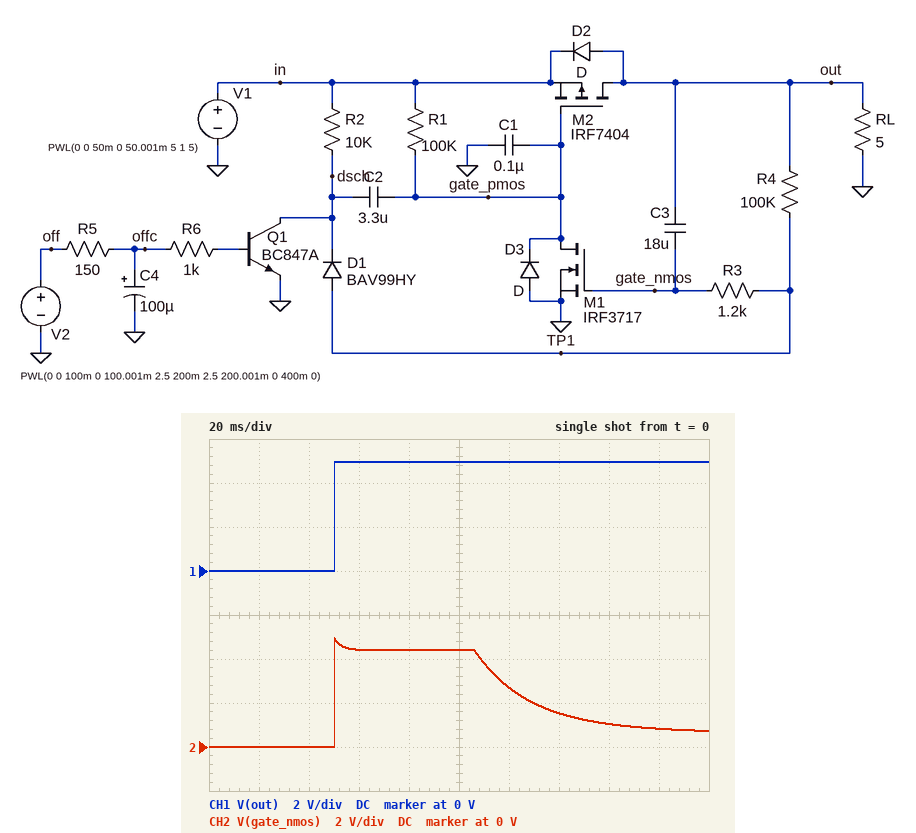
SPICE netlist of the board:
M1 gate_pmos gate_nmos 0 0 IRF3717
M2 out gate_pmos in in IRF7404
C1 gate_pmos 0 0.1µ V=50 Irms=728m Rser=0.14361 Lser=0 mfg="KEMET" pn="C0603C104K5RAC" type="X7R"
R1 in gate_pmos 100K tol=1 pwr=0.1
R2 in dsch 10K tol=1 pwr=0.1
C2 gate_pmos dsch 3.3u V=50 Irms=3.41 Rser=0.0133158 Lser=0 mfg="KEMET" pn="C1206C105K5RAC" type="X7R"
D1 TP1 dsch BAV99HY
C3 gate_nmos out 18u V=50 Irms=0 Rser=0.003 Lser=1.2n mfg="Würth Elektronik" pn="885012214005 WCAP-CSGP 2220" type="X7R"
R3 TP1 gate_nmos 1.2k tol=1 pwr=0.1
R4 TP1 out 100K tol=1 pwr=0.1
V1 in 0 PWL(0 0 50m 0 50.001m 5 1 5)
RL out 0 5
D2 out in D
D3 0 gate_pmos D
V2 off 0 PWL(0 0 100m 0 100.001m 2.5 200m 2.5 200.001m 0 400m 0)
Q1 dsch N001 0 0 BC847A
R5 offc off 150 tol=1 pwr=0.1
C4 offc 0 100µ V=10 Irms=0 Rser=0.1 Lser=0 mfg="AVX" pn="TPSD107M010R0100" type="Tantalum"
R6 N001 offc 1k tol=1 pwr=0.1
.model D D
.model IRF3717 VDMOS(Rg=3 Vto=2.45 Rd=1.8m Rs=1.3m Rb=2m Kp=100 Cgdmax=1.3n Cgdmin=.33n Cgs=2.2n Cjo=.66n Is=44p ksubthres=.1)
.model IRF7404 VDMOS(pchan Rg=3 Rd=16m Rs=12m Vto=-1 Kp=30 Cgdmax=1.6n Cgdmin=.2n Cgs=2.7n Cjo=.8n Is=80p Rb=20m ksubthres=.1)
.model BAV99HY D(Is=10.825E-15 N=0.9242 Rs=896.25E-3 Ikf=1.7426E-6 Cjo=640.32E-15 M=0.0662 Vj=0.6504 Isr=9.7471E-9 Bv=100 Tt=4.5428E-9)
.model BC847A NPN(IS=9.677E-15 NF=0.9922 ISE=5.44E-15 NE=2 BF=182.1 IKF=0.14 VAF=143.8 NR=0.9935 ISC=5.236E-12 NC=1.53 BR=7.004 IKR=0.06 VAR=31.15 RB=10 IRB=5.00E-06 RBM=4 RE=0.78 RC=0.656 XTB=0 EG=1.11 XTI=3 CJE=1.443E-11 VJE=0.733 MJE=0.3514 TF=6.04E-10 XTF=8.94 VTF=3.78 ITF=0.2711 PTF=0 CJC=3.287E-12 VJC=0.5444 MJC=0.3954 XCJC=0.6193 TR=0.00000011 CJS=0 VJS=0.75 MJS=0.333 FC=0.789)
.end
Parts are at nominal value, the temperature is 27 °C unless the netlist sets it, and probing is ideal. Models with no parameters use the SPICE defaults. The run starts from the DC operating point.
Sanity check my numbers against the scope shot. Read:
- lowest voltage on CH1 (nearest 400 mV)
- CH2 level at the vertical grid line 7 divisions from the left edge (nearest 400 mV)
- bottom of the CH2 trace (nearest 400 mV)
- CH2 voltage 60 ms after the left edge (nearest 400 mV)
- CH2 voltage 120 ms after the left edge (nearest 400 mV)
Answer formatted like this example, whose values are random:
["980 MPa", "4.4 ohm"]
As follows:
["0 V", "1.6 V", "0 V", "4.4 V", "2.8 V"]
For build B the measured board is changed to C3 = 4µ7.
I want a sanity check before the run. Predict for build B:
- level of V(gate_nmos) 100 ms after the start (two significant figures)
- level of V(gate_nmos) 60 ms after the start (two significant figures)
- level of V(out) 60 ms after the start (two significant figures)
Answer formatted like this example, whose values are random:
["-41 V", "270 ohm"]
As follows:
["3.6 V", "3.5 V", "5.0 V"]
